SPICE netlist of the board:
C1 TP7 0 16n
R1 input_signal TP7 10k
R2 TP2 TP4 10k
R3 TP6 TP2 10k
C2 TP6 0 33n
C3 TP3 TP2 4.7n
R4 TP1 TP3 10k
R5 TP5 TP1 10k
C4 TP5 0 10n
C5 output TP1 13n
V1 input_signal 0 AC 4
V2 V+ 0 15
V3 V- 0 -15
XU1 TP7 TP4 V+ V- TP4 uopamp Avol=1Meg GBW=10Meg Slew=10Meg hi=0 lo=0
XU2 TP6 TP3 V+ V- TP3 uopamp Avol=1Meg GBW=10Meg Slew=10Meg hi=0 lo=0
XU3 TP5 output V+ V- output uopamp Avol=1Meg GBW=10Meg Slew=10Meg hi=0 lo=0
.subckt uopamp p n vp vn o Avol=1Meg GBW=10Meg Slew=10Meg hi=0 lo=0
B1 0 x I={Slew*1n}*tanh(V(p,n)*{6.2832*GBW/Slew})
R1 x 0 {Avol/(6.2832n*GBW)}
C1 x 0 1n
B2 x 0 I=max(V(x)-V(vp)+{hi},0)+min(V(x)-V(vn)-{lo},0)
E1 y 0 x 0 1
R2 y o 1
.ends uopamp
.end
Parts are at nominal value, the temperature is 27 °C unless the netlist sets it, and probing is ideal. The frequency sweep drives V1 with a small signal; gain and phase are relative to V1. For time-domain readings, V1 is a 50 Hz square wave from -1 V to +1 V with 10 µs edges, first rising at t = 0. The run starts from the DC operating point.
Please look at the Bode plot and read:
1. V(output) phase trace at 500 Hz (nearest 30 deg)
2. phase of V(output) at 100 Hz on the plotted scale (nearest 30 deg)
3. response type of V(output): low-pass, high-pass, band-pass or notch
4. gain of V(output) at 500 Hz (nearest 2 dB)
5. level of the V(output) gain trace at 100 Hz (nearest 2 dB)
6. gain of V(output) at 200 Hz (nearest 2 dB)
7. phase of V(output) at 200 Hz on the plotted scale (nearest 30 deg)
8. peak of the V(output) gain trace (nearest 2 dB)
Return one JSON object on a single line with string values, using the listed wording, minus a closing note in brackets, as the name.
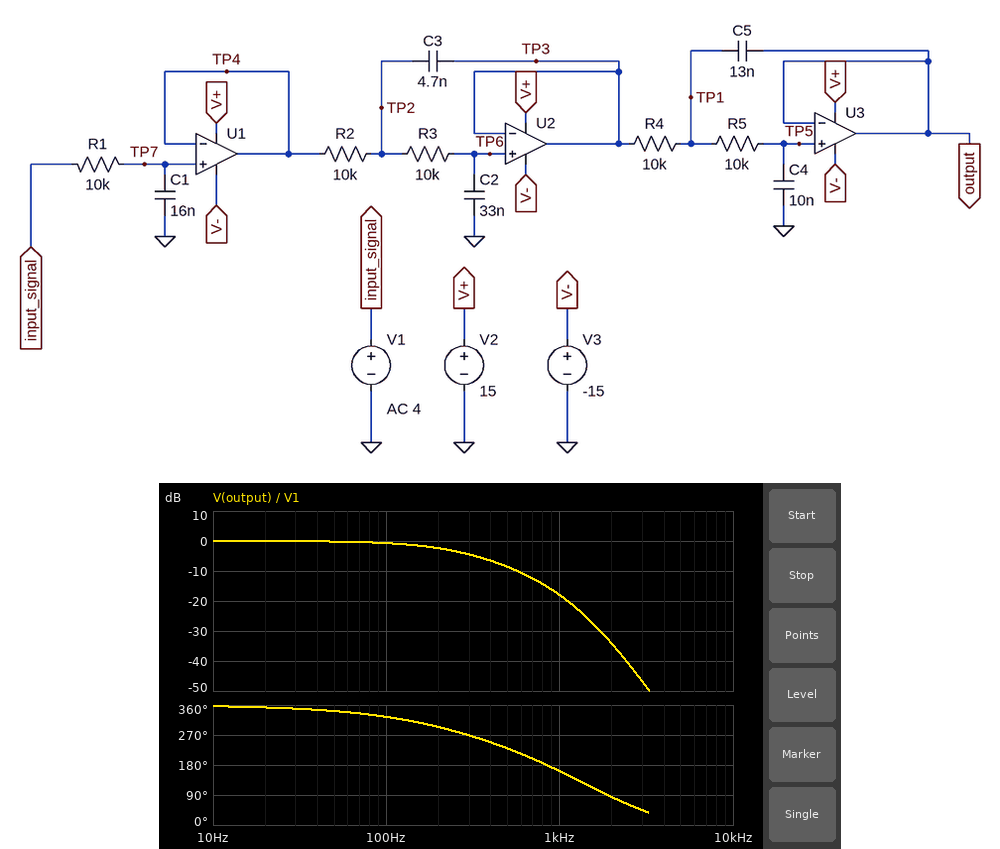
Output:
{"V(output) phase trace at 500 Hz": "240 deg", "phase of V(output) at 100 Hz on the plotted scale": "330 deg", "response type of V(output): low-pass, high-pass, band-pass or notch": "low-pass", "gain of V(output) at 500 Hz": "-8 dB", "level of the V(output) gain trace at 100 Hz": "0 dB", "gain of V(output) at 200 Hz": "-2 dB", "phase of V(output) at 200 Hz on the plotted scale": "300 deg", "peak of the V(output) gain trace": "0 dB"}
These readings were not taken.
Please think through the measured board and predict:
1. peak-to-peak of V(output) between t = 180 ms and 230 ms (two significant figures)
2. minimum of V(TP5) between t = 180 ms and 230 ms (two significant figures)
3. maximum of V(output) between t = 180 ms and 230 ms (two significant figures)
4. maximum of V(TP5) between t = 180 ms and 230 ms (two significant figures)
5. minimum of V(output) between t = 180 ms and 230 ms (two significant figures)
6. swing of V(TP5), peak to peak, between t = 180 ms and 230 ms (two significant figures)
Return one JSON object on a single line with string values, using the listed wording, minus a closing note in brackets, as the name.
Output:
{"peak-to-peak of V(output) between t = 180 ms and 230 ms": "2.0 V", "minimum of V(TP5) between t = 180 ms and 230 ms": "-1.0 V", "maximum of V(output) between t = 180 ms and 230 ms": "1.0 V", "maximum of V(TP5) between t = 180 ms and 230 ms": "1.0 V", "minimum of V(output) between t = 180 ms and 230 ms": "-1.0 V", "swing of V(TP5), peak to peak, between t = 180 ms and 230 ms": "2.0 V"}
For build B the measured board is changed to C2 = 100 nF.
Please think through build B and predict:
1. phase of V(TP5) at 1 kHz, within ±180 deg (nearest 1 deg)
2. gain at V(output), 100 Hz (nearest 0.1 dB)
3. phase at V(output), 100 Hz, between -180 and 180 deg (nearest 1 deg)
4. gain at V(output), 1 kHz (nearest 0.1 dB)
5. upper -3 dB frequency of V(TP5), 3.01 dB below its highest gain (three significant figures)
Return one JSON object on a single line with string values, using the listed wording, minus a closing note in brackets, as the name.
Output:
{"phase of V(TP5) at 1 kHz, within ±180 deg": "152 deg", "gain at V(output), 100 Hz": "-4.1 dB", "phase at V(output), 100 Hz, between -180 and 180 deg": "-65 deg", "gain at V(output), 1 kHz": "-27.6 dB", "upper -3 dB frequency of V(TP5), 3.01 dB below its highest gain": "79.7 Hz"}
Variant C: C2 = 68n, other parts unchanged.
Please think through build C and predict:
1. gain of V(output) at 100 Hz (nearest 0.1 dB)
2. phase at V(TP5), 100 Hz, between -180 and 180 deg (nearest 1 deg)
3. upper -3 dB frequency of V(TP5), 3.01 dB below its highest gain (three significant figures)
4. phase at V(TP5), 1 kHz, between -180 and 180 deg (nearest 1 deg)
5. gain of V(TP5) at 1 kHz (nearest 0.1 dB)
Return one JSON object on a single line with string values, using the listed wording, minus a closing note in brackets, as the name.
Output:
{"gain of V(output) at 100 Hz": "-2.4 dB", "phase at V(TP5), 100 Hz, between -180 and 180 deg": "-54 deg", "upper -3 dB frequency of V(TP5), 3.01 dB below its highest gain": "117 Hz", "phase at V(TP5), 1 kHz, between -180 and 180 deg": "154 deg", "gain of V(TP5) at 1 kHz": "-24.3 dB"}
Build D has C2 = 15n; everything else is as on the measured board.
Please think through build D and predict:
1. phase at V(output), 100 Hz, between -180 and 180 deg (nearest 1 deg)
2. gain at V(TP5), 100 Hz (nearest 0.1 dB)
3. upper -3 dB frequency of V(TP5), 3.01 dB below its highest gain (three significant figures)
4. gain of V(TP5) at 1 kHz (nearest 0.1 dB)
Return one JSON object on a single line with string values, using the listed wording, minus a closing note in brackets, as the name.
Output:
{"phase at V(output), 100 Hz, between -180 and 180 deg": "-24 deg", "gain at V(TP5), 100 Hz": "-0.2 dB", "upper -3 dB frequency of V(TP5), 3.01 dB below its highest gain": "421 Hz", "gain of V(TP5) at 1 kHz": "-11.7 dB"}
